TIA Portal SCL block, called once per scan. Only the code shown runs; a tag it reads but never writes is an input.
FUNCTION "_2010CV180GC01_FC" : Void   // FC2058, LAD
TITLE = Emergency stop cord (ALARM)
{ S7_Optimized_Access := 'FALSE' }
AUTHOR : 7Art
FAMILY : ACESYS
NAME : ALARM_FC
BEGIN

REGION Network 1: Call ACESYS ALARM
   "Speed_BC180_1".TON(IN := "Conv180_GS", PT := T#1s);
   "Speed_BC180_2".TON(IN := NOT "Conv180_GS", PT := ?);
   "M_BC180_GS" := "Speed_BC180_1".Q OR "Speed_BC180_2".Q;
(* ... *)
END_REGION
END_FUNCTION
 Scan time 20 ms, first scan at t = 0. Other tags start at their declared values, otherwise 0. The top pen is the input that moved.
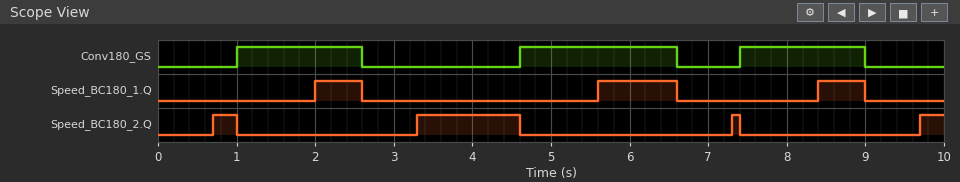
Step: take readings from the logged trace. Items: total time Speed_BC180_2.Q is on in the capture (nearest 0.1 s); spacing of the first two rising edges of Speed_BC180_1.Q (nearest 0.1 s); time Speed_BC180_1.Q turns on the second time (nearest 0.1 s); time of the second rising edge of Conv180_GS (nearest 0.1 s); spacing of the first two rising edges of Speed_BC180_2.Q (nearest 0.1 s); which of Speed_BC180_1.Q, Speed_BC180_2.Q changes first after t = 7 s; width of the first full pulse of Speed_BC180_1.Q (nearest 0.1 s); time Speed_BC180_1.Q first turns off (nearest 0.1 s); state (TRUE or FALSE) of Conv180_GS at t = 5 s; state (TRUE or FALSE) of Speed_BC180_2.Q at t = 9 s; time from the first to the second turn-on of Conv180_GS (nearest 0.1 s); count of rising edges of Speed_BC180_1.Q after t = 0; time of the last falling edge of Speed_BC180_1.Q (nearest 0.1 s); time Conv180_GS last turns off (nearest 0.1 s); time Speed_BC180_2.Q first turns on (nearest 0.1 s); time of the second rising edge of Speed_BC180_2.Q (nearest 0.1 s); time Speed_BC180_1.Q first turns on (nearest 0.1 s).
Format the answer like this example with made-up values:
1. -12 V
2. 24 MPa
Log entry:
1. 2.0 s
2. 3.6 s
3. 5.6 s
4. 4.6 s
5. 2.6 s
6. Speed_BC180_2.Q
7. 0.6 s
8. 2.6 s
9. TRUE
10. FALSE
11. 3.6 s
12. 3
13. 9.0 s
14. 9.0 s
15. 0.7 s
16. 3.3 s
17. 2.0 s
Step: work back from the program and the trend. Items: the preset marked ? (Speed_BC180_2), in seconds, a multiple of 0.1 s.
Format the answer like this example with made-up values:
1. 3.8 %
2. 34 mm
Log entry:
1. 0.7 s
